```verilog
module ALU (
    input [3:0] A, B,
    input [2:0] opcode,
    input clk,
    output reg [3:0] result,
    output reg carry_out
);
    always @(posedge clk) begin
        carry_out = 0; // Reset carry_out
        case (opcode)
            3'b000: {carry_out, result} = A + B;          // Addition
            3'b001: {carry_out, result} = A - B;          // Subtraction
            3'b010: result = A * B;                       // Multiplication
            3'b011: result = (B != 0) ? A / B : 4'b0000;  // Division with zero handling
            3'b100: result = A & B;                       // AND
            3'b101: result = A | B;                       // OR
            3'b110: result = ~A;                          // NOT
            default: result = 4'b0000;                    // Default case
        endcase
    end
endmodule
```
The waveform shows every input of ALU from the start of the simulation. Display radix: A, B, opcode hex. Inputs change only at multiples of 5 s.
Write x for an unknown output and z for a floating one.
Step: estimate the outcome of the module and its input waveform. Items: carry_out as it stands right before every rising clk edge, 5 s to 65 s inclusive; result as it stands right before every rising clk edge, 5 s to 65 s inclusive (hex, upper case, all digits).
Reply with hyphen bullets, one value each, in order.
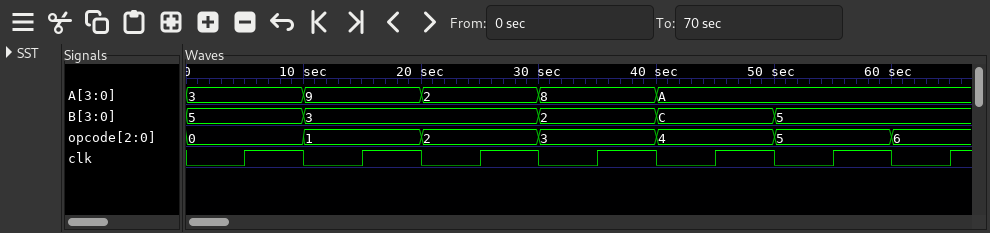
- x 0 0 0 0 0 0
- x, 8, 6, 6, 4, 8, F
